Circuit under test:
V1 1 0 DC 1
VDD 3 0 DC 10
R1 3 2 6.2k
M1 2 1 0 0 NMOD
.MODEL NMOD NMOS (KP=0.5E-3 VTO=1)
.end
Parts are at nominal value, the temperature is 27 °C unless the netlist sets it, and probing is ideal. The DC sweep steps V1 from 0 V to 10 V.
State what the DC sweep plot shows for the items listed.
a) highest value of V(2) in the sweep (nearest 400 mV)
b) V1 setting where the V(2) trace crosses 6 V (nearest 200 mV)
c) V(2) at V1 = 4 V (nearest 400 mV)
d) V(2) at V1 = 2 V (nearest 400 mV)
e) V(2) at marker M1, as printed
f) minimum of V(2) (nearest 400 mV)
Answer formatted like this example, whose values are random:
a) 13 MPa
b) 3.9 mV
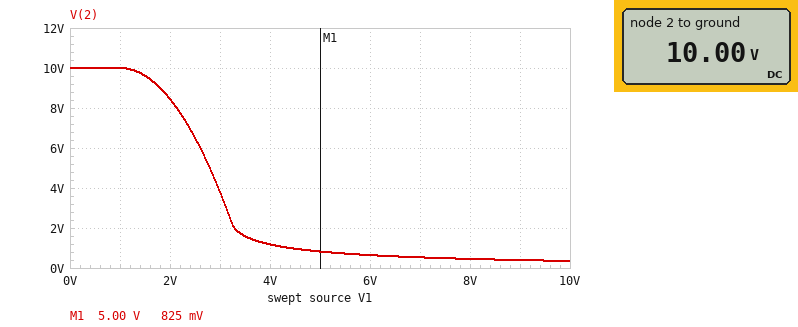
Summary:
a) 10.0 V
b) 2.6 V
c) 1.2 V
d) 8.4 V
e) 825 mV
f) 400 mV
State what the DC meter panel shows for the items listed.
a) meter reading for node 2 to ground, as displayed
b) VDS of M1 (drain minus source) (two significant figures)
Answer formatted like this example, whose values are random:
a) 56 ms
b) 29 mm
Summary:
a) 10.00 V
b) 10 V
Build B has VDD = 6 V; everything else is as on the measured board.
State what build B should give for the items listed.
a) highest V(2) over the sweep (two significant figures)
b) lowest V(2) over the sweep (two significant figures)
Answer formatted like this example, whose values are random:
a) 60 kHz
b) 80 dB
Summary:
a) 6.0 V
b) 210 mV
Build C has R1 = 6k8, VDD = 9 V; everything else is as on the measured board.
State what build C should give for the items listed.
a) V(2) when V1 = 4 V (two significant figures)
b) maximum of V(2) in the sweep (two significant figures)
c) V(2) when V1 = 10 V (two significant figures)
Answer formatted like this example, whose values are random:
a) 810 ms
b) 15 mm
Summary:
a) 940 mV
b) 9.0 V
c) 290 mV
